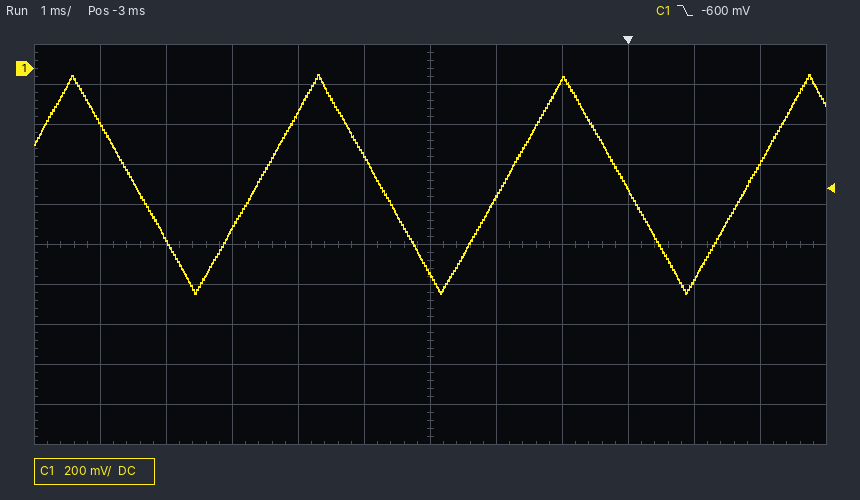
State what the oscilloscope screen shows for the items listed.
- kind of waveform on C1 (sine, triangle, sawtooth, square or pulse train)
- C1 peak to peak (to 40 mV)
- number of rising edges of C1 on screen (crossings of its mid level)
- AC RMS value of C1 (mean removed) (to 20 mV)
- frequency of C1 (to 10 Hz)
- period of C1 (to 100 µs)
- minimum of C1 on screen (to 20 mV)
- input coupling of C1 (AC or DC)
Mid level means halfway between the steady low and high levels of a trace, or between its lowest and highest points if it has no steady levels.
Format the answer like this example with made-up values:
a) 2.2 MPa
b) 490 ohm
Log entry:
a) triangle
b) 1.08 V
c) 3
d) 320 mV
e) 270 Hz
f) 3.7 ms
g) -1.12 V
h) DC
